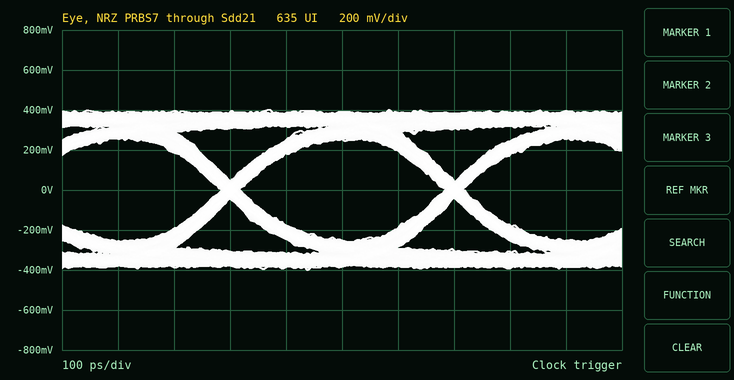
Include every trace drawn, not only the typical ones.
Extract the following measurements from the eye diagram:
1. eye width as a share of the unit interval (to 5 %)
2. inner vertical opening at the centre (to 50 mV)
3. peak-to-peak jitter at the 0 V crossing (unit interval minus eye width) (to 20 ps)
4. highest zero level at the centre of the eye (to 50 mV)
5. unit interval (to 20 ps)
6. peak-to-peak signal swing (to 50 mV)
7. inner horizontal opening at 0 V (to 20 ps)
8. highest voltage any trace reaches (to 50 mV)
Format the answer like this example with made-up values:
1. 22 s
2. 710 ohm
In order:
1. 90 %
2. 500 mV
3. 40 ps
4. -250 mV
5. 400 ps
6. 800 mV
7. 360 ps
8. 400 mV
